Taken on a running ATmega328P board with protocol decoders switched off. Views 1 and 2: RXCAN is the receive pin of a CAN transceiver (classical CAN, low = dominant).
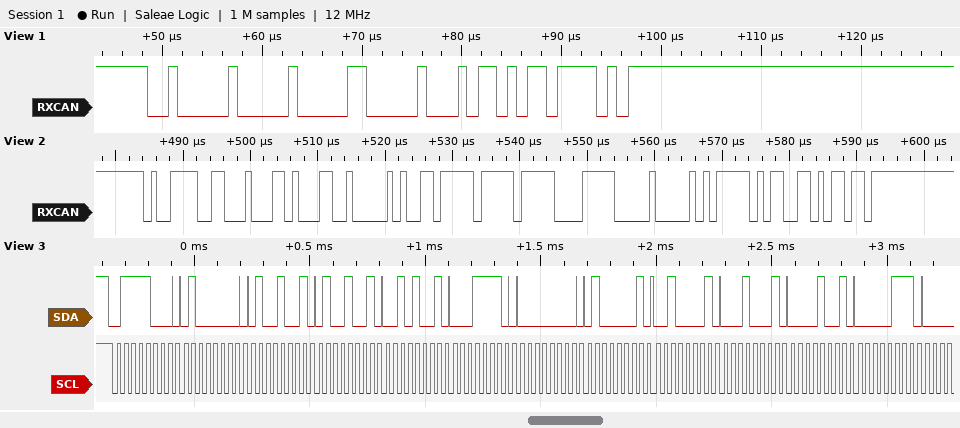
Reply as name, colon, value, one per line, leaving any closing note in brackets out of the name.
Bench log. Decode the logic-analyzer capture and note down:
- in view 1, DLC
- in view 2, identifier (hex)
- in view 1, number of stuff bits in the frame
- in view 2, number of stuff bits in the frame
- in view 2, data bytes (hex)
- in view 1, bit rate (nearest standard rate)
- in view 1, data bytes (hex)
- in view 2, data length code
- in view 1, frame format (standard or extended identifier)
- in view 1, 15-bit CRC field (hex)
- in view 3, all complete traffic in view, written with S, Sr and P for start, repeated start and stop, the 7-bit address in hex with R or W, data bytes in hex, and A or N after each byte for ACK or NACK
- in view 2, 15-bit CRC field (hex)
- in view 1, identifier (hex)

in view 1, DLC: 1
in view 2, identifier: 0x4F3
in view 1, number of stuff bits in the frame: 4
in view 2, number of stuff bits in the frame: 8
in view 2, data bytes: D1 90 26 FF FE 3E 00 5F
in view 1, bit rate: 1000 kbit/s
in view 1, data bytes: 00
in view 2, data length code: 8
in view 1, frame format: standard
in view 1, 15-bit CRC field: 0x5ADE
in view 3, all complete traffic in view, written with S, Sr and P for start, repeated start and stop, the 7-bit address in hex with R or W, data bytes in hex, and A or N after each byte for ACK or NACK: S 3CW A 40 A 49 A 49 A 29 A 1E A 00 A 41 A 21 A 11 A 09 A 07 A
in view 2, 15-bit CRC field: 0x59AD
in view 1, identifier: 0x200
